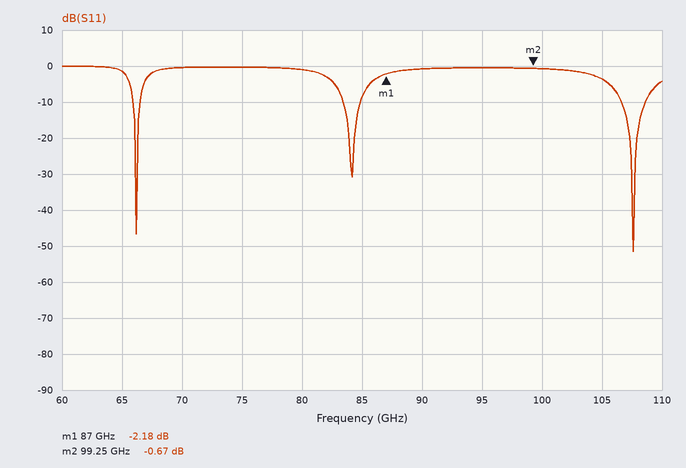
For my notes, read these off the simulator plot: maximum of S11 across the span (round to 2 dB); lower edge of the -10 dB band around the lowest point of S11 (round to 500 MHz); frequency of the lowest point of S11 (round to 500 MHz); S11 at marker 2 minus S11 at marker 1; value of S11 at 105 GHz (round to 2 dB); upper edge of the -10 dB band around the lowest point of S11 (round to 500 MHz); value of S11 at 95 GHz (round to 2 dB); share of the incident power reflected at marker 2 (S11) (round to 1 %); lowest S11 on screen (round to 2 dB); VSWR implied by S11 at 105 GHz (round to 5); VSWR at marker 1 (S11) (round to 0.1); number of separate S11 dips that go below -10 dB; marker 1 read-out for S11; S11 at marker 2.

0 dB
106.5 GHz
107.5 GHz
1.51 dB
-4 dB
108.5 GHz
0 dB
86 %
-52 dB
5
8.0
3
-2.18 dB
-0.67 dB
